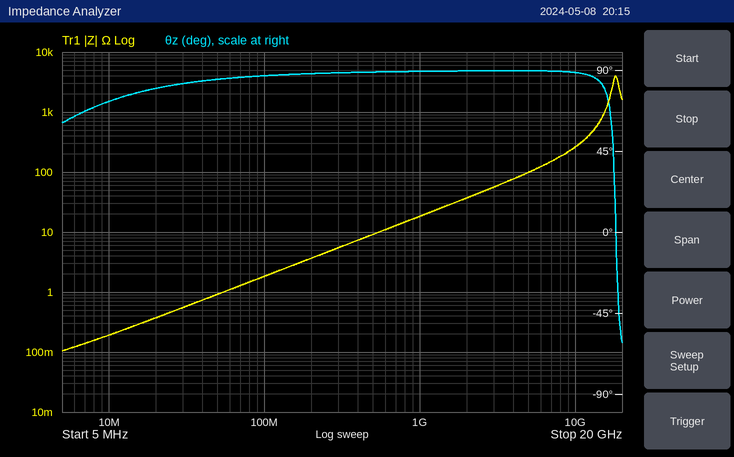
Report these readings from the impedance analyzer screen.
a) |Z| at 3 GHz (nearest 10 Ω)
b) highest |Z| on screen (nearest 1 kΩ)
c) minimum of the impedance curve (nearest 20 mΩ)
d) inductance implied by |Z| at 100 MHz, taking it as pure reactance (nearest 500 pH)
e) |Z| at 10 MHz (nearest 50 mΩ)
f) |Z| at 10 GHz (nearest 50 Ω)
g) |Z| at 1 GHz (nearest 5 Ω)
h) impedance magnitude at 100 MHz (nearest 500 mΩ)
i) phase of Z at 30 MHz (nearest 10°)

60 Ω
4 kΩ
100 mΩ
3.0 nH
200 mΩ
250 Ω
20 Ω
2.0 Ω
80°
